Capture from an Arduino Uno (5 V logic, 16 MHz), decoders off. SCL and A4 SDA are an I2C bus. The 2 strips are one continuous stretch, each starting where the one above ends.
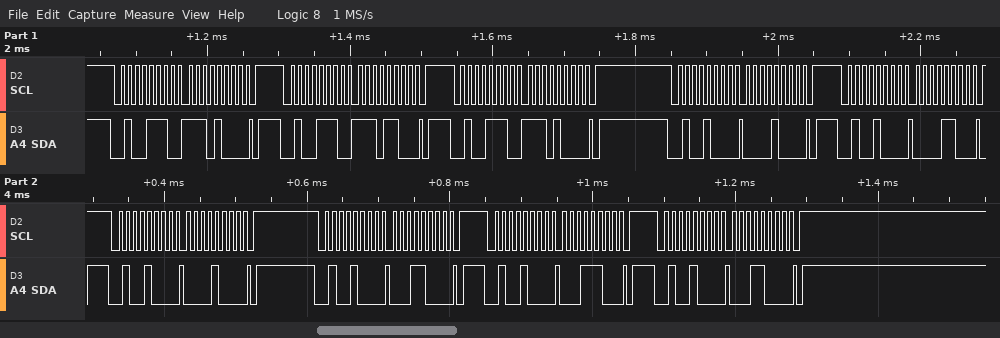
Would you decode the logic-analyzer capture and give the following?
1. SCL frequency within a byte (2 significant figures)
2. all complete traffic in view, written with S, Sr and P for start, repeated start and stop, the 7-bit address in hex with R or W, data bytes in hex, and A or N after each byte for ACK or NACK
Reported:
100 kHz
S 27W A E8 A P S 27W A EC A P S 27W A E8 A P S 24W A 08 A P S 24W A 0C A P S 24W A 08 A P S 24W A 18 A P S 24W A 1C A P S 24W A 18 A P
